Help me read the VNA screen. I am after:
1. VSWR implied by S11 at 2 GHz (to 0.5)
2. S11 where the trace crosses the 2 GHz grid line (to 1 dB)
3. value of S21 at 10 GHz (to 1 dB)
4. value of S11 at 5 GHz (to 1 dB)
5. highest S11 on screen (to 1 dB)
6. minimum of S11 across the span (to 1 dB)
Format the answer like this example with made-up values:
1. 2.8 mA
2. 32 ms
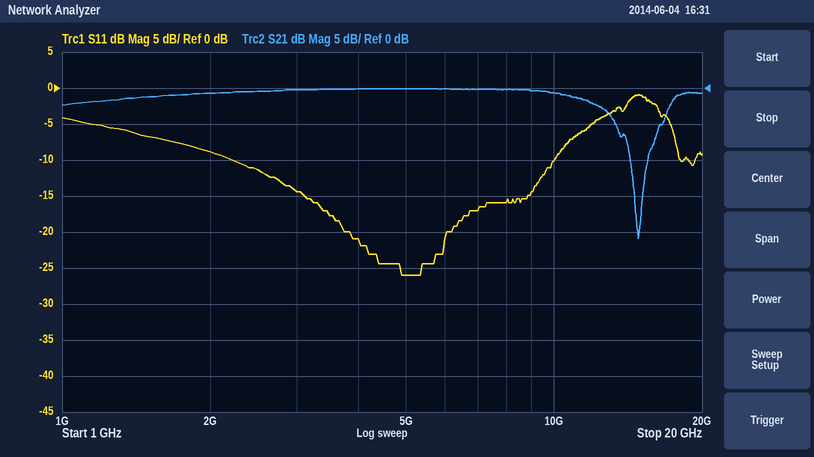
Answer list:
1. 2.0
2. -9 dB
3. -1 dB
4. -26 dB
5. -1 dB
6. -26 dB
